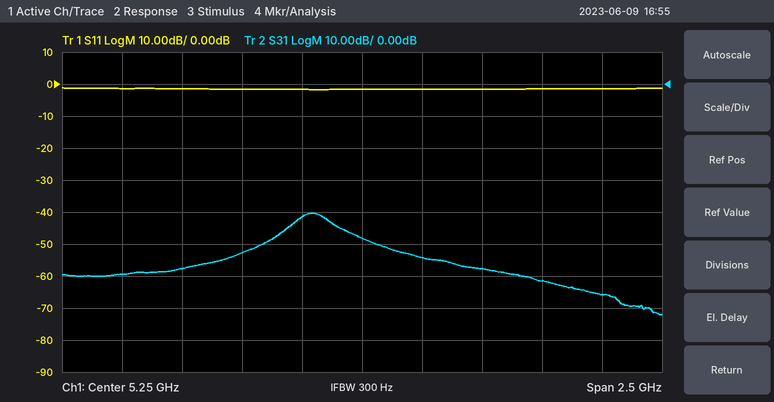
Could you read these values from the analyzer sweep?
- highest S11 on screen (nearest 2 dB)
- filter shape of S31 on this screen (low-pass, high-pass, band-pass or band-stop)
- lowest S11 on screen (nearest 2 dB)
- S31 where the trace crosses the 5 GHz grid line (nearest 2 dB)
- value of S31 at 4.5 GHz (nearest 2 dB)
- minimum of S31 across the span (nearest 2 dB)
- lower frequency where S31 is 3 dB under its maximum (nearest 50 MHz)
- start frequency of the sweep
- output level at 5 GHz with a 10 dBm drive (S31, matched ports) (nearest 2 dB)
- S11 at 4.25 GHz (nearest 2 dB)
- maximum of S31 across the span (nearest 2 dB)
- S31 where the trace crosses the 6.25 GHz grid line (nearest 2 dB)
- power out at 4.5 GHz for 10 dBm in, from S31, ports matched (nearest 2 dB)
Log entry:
-2 dB
band-pass
-2 dB
-42 dB
-58 dB
-72 dB
4.95 GHz
4 GHz
-32 dBm
-2 dB
-40 dB
-66 dB
-48 dBm
